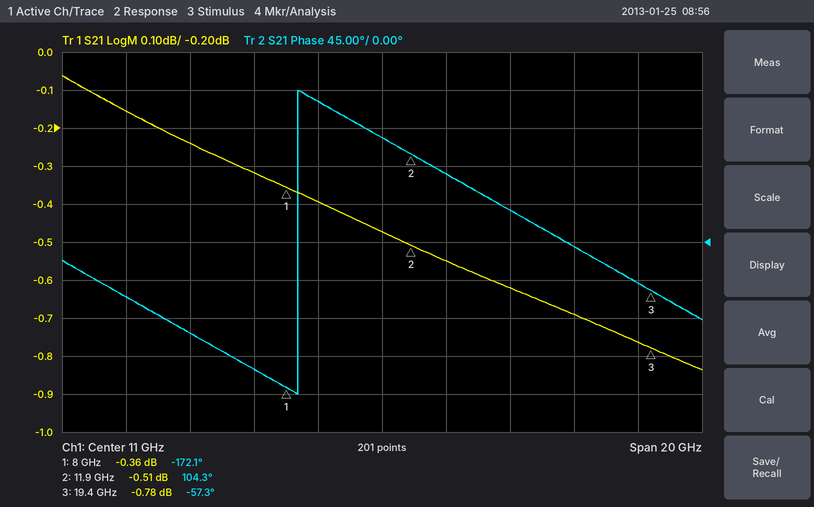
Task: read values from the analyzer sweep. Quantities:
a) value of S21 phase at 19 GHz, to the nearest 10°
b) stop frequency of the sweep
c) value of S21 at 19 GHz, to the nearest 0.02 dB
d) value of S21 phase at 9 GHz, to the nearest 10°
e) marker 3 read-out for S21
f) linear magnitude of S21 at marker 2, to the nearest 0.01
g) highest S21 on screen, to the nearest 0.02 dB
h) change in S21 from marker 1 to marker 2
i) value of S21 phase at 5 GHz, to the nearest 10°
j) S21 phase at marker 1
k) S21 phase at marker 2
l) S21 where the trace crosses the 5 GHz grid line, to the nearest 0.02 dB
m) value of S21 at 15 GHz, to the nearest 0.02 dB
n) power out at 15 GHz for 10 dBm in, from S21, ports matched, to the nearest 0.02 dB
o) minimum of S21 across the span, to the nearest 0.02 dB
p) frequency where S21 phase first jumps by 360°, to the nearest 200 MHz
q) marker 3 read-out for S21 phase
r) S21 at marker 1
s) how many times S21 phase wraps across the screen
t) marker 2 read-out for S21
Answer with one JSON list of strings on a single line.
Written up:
["-50°", "21 GHz", "-0.76 dB", "170°", "-0.78 dB", "0.94", "-0.06 dB", "-0.15 dB", "-110°", "-172.1°", "104.3°", "-0.24 dB", "-0.62 dB", "9.38 dBm", "-0.84 dB", "8.4 GHz", "-57.3°", "-0.36 dB", "1", "-0.51 dB"]
